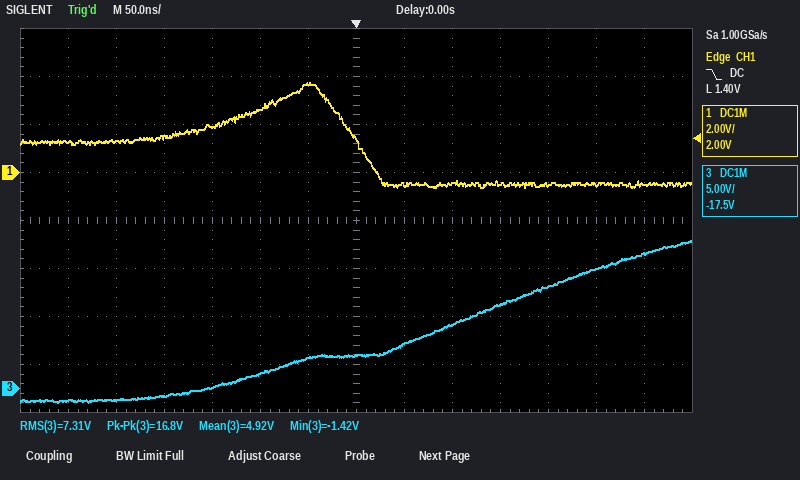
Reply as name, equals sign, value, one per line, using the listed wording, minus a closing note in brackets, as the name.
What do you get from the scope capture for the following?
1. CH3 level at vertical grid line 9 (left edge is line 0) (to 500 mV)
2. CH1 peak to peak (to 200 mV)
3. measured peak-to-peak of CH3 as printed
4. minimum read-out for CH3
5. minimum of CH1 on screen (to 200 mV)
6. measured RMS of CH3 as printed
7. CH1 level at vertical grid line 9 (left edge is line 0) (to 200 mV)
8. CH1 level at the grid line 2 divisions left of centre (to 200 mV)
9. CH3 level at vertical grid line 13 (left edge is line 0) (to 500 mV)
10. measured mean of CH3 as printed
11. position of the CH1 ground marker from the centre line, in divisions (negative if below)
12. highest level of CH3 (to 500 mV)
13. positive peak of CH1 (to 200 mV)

CH3 level at vertical grid line 9 (left edge is line 0) = 6.5 V
CH1 peak to peak = 4.4 V
measured peak-to-peak of CH3 as printed = 16.8 V
minimum read-out for CH3 = -1.42 V
minimum of CH1 on screen = -600 mV
measured RMS of CH3 as printed = 7.31 V
CH1 level at vertical grid line 9 (left edge is line 0) = -400 mV
CH1 level at the grid line 2 divisions left of centre = 2.6 V
CH3 level at vertical grid line 13 (left edge is line 0) = 14.0 V
measured mean of CH3 as printed = 4.92 V
position of the CH1 ground marker from the centre line, in divisions = +1.0 div
highest level of CH3 = 15.5 V
positive peak of CH1 = 3.8 V
